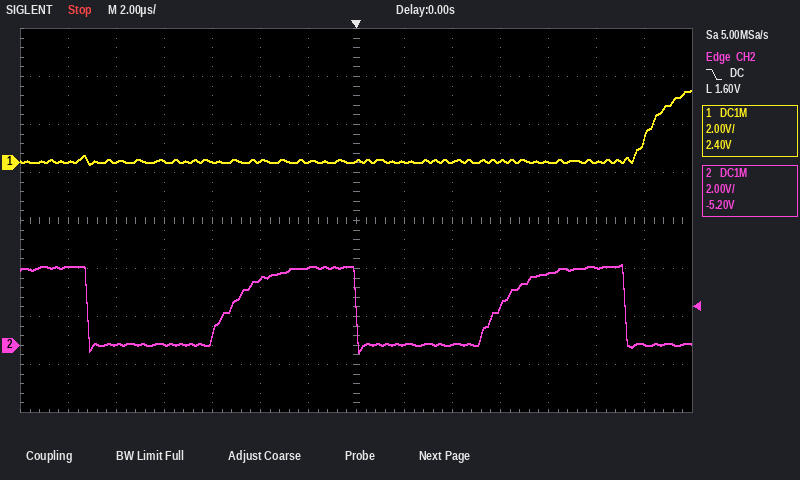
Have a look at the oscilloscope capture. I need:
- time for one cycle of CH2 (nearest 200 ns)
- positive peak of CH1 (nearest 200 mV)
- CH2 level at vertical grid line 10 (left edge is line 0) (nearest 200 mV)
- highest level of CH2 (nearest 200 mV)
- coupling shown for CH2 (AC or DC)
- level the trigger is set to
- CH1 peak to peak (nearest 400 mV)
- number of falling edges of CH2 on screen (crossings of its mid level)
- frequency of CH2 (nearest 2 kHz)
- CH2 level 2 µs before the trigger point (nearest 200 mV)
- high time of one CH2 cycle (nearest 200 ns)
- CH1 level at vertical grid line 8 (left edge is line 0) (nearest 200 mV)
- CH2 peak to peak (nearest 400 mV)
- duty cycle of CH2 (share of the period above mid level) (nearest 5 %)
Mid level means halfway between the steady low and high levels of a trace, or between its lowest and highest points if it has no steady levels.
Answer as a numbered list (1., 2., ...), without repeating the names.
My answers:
1. 11.2 µs
2. 3.0 V
3. 1.6 V
4. 3.4 V
5. DC
6. 1.60 V
7. 3.2 V
8. 3
9. 90 kHz
10. 3.2 V
11. 5.2 µs
12. 0.0 V
13. 3.6 V
14. 45 %
